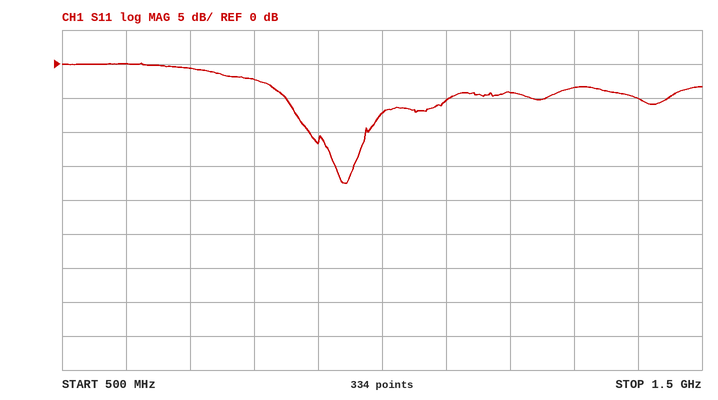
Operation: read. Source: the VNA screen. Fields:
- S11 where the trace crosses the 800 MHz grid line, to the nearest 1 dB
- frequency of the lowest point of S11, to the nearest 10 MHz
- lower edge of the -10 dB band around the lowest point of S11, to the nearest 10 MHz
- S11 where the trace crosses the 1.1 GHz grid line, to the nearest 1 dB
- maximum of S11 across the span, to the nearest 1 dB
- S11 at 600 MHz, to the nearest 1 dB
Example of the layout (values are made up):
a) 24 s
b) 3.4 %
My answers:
a) -2 dB
b) 940 MHz
c) 890 MHz
d) -5 dB
e) 0 dB
f) 0 dB
